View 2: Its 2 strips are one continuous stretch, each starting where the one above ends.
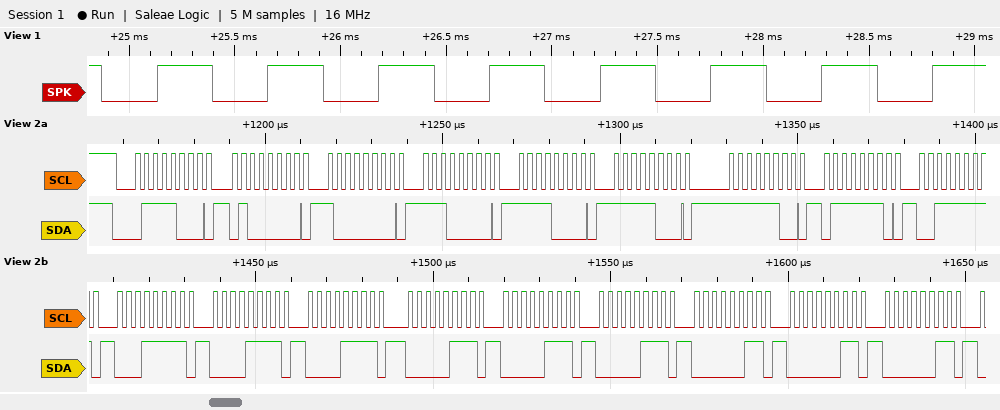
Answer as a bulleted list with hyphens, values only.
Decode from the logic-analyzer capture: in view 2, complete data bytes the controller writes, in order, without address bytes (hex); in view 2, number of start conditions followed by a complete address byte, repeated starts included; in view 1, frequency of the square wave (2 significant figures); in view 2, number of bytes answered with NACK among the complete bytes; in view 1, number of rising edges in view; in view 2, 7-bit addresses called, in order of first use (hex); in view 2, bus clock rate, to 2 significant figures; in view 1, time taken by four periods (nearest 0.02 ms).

- 40 80 E0 F0 F8 FC 7E 3F 1F 0F 0F 07 07 07 03 03 03
- 1
- 1.9 kHz
- 0
- 8
- 0x3C
- 400 kHz
- 2.10 ms
